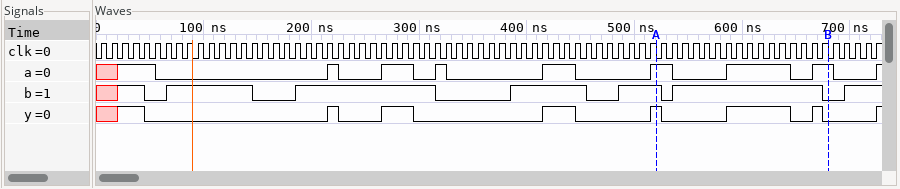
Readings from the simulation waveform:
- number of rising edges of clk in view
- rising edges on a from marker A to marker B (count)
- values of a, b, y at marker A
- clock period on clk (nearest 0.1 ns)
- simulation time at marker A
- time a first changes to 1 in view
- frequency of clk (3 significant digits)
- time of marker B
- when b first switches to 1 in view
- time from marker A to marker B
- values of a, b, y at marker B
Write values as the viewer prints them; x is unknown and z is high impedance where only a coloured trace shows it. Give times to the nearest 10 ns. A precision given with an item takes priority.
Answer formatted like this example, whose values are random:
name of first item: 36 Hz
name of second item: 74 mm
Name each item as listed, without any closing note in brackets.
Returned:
number of rising edges of clk in view: 73
rising edges on a from marker A to marker B: 2
values of a, b, y at marker A: a=1, b=1, y=1
clock period on clk: 10 ns
simulation time at marker A: 520 ns
time a first changes to 1 in view: 20 ns
frequency of clk: 100 MHz
time of marker B: 680 ns
when b first switches to 1 in view: 20 ns
time from marker A to marker B: 160 ns
values of a, b, y at marker B: a=1, b=0, y=0
